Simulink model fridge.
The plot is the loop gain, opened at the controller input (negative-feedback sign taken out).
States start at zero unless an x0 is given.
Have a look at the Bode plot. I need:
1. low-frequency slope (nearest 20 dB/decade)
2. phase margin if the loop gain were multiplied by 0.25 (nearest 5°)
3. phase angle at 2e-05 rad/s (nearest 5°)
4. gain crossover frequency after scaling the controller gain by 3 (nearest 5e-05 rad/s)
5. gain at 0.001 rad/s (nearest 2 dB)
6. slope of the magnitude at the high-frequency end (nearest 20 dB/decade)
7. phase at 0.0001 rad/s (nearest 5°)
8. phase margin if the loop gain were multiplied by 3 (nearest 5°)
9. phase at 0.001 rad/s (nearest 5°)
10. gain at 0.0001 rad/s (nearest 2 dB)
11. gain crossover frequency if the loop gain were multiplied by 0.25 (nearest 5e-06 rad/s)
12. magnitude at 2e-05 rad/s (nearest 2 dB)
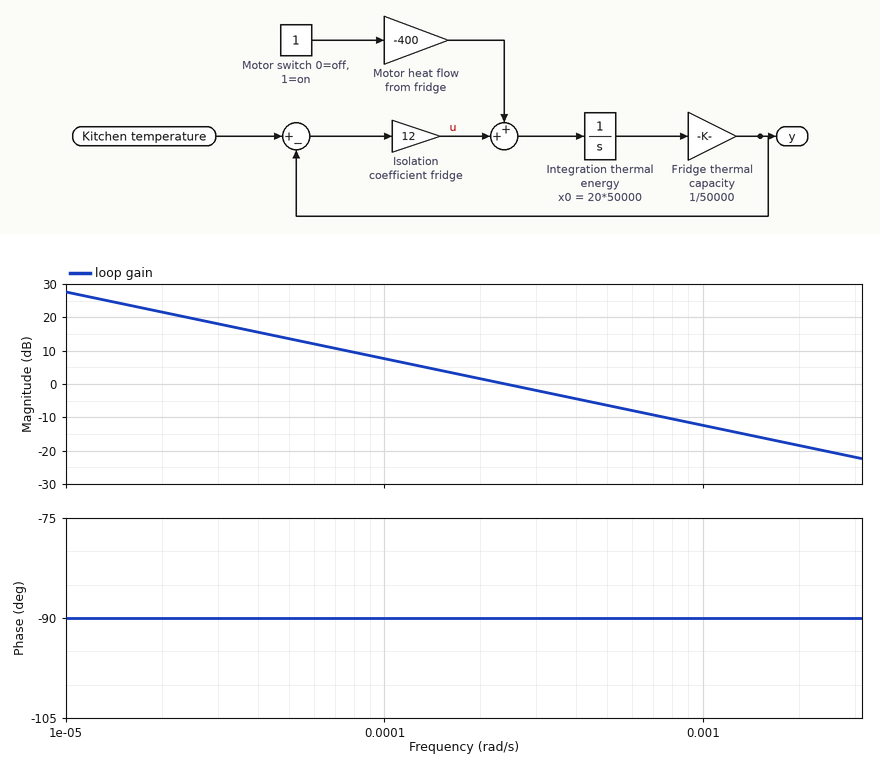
-20 dB/decade
90°
-90°
0.00070 rad/s
-12 dB
-20 dB/decade
-90°
90°
-90°
8 dB
0.000060 rad/s
22 dB
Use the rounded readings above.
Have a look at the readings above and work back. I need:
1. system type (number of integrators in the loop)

1
